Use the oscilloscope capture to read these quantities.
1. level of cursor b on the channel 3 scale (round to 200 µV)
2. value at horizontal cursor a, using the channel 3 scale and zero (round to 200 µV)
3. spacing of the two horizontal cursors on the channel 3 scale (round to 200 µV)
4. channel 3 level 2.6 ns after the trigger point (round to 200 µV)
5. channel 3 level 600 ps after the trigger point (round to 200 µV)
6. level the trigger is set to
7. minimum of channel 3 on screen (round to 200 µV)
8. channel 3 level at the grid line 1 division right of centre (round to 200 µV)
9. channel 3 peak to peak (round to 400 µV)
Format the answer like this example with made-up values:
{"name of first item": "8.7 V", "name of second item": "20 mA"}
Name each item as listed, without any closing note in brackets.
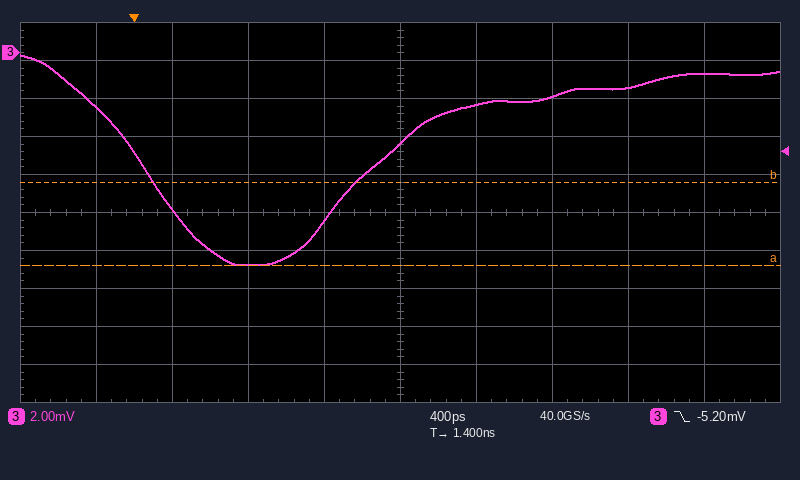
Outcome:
{"level of cursor b on the channel 3 scale": "-6.8 mV", "value at horizontal cursor a, using the channel 3 scale and zero": "-11.2 mV", "spacing of the two horizontal cursors on the channel 3 scale": "4.4 mV", "channel 3 level 2.6 ns after the trigger point": "-1.8 mV", "channel 3 level 600 ps after the trigger point": "-11.2 mV", "level the trigger is set to": "-5.20 mV", "minimum of channel 3 on screen": "-11.2 mV", "channel 3 level at the grid line 1 division right of centre": "-2.8 mV", "channel 3 peak to peak": "11.2 mV"}
